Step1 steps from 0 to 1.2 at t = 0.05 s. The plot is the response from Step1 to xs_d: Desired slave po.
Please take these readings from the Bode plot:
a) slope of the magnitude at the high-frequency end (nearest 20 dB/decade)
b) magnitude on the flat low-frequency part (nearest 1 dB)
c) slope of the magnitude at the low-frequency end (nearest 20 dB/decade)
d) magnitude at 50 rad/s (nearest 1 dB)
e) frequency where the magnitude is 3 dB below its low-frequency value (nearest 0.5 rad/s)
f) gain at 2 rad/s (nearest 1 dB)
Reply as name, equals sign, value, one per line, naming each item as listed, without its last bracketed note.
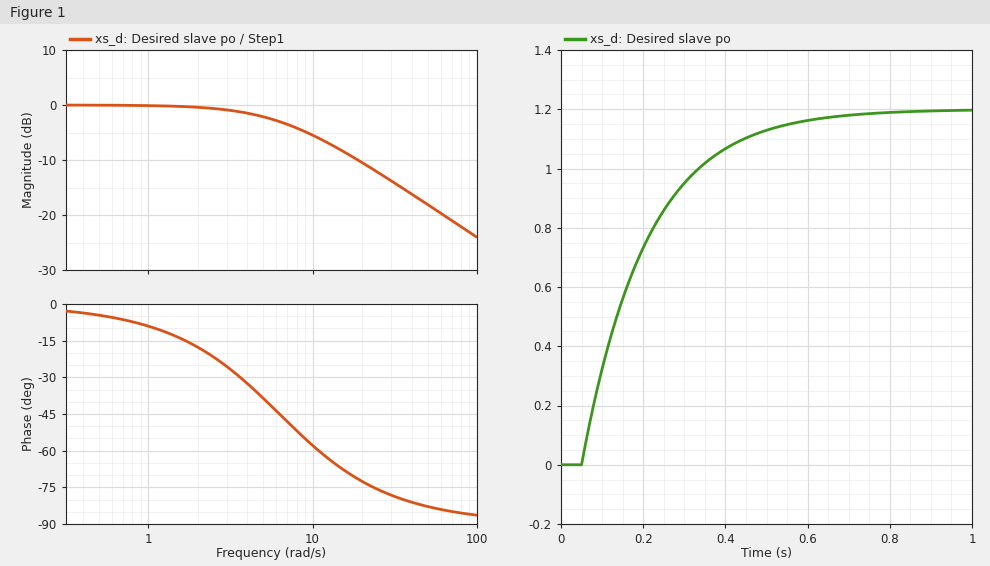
slope of the magnitude at the high-frequency end = -20 dB/decade
magnitude on the flat low-frequency part = 0 dB
slope of the magnitude at the low-frequency end = 0 dB/decade
magnitude at 50 rad/s = -18 dB
frequency where the magnitude is 3 dB below its low-frequency value = 6.5 rad/s
gain at 2 rad/s = 0 dB
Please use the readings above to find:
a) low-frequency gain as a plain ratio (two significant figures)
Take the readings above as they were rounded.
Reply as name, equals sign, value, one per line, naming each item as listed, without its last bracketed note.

low-frequency gain as a plain ratio = 1.0
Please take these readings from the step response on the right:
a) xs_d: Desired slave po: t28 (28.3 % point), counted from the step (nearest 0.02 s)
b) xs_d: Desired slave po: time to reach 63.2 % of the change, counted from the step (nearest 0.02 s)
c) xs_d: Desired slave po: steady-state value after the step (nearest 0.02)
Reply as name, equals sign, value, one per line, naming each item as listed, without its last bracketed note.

xs_d: Desired slave po: t28 (28.3 % point), counted from the step = 0.06 s
xs_d: Desired slave po: time to reach 63.2 % of the change, counted from the step = 0.16 s
xs_d: Desired slave po: steady-state value after the step = 1.20
